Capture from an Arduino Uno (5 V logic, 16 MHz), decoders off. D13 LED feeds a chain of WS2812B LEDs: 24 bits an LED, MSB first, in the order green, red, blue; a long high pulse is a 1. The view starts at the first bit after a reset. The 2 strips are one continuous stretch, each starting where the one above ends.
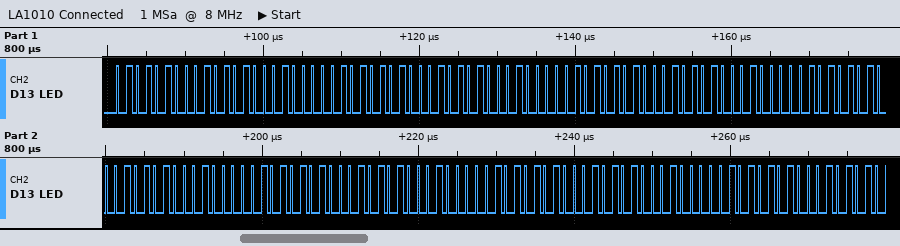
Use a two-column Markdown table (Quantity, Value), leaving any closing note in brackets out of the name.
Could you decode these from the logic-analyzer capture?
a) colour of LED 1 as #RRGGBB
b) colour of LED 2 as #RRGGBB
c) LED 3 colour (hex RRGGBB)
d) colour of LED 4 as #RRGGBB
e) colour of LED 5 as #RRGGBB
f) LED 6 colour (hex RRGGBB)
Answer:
| Quantity | Value |
|---|---|
| colour of LED 1 as #RRGGBB | #545441 |
| colour of LED 2 as #RRGGBB | #545441 |
| LED 3 colour | #545441 |
| colour of LED 4 as #RRGGBB | #545441 |
| colour of LED 5 as #RRGGBB | #545441 |
| LED 6 colour | #545441 |
